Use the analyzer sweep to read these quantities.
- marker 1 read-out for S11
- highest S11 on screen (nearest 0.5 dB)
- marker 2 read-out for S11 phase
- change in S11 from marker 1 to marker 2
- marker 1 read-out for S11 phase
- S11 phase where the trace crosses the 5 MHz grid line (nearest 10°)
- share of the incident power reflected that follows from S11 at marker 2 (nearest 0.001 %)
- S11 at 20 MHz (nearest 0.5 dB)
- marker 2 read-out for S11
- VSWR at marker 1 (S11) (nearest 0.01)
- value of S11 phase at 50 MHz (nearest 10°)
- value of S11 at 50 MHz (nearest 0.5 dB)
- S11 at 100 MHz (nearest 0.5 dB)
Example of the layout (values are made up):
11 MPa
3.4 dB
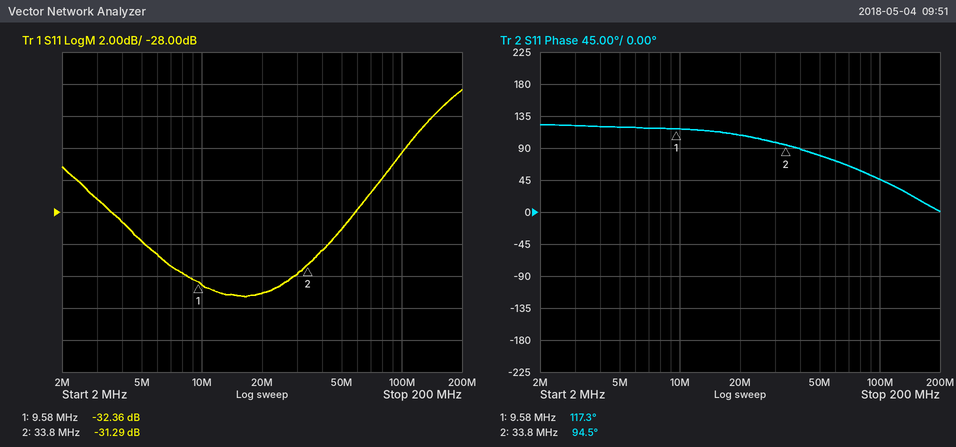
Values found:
-32.36 dB
-20.5 dB
94.5°
1.07 dB
117.3°
120°
0.074 %
-33.0 dB
-31.29 dB
1.05
80°
-29.0 dB
-24.5 dB
